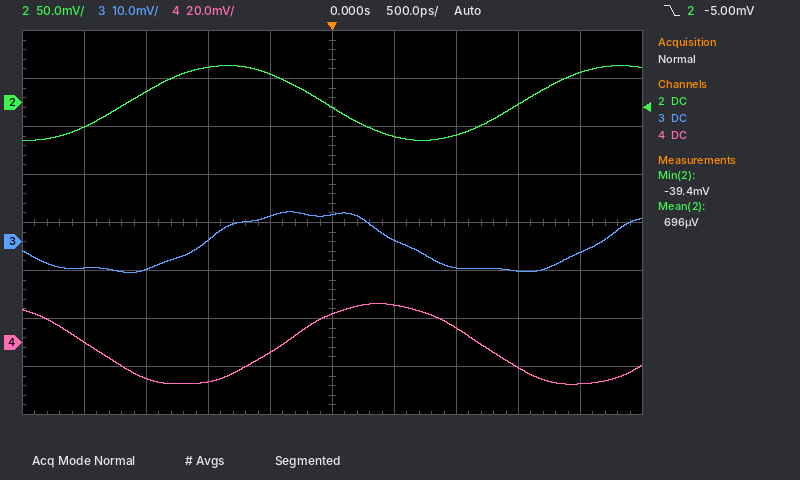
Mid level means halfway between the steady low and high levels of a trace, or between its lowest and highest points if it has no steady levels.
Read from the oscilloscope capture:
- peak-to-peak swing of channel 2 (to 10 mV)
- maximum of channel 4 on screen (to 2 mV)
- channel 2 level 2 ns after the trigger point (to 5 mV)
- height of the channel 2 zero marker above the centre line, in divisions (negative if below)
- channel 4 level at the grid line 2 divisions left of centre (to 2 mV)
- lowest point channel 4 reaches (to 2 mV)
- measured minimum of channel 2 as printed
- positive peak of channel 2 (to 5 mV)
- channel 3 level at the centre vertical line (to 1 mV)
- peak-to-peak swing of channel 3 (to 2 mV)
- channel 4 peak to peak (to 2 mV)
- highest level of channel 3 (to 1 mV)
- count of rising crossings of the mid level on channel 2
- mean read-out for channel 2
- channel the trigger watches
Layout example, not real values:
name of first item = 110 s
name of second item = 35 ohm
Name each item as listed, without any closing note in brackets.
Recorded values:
peak-to-peak swing of channel 2 = 80 mV
maximum of channel 4 on screen = 16 mV
channel 2 level 2 ns after the trigger point = 30 mV
height of the channel 2 zero marker above the centre line, in divisions = +2.5 div
channel 4 level at the grid line 2 divisions left of centre = -16 mV
lowest point channel 4 reaches = -18 mV
measured minimum of channel 2 as printed = -39.4 mV
positive peak of channel 2 = 40 mV
channel 3 level at the centre vertical line = 6 mV
peak-to-peak swing of channel 3 = 12 mV
channel 4 peak to peak = 34 mV
highest level of channel 3 = 6 mV
count of rising crossings of the mid level on channel 2 = 2
mean read-out for channel 2 = 696 µV
channel the trigger watches = channel 2
